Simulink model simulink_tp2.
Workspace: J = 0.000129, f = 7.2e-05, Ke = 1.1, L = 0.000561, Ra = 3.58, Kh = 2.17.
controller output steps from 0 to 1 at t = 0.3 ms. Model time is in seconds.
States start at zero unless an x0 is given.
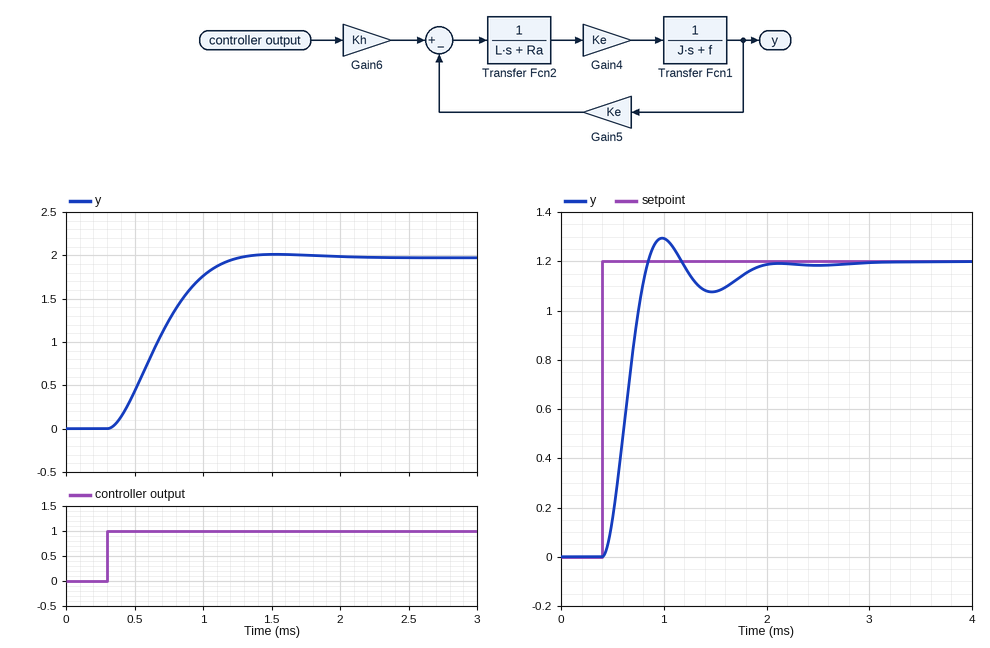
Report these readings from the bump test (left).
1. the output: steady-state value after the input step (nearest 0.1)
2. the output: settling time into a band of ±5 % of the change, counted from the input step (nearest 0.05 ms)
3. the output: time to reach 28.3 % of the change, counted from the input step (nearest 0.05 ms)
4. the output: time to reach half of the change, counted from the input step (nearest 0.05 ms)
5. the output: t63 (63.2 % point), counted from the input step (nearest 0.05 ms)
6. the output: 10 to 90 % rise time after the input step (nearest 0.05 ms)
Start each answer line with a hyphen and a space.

- 2.0
- 0.80 ms
- 0.25 ms
- 0.35 ms
- 0.45 ms
- 0.60 ms
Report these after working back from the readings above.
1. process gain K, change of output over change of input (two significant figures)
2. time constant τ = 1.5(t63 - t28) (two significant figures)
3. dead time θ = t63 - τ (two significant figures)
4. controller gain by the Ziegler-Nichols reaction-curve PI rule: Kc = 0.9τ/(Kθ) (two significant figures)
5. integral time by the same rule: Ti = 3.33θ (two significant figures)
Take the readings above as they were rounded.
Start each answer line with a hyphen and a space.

- 2.0
- 0.30 ms
- 0.15 ms
- 0.90
- 0.50 ms
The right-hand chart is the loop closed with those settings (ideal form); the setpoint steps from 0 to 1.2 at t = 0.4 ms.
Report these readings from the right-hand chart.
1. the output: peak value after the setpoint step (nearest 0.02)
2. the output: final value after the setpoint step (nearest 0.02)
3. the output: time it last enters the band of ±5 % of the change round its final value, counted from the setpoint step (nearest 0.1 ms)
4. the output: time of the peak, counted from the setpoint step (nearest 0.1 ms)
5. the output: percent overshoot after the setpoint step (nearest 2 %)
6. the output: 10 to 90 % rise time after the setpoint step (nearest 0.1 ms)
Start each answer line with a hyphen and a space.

- 1.30
- 1.20
- 1.4 ms
- 0.6 ms
- 8 %
- 0.3 ms
